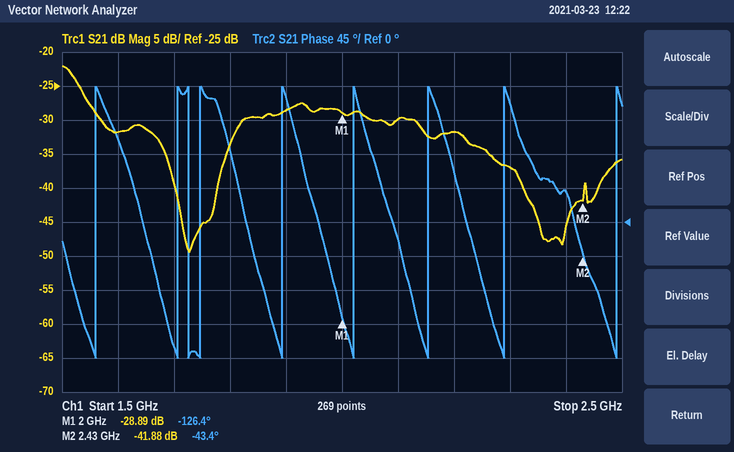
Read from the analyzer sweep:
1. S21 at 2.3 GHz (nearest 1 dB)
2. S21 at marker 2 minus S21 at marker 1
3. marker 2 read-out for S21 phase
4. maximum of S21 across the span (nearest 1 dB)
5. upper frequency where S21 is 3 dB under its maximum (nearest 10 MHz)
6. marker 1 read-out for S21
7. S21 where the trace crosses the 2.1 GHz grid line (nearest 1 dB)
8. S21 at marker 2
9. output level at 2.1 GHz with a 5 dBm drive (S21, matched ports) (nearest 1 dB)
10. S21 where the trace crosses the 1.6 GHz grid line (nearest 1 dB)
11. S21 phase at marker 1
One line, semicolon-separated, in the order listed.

-37 dB; -12.99 dB; -43.4°; -22 dB; 1.53 GHz; -28.89 dB; -30 dB; -41.88 dB; -25 dBm; -32 dB; -126.4°
